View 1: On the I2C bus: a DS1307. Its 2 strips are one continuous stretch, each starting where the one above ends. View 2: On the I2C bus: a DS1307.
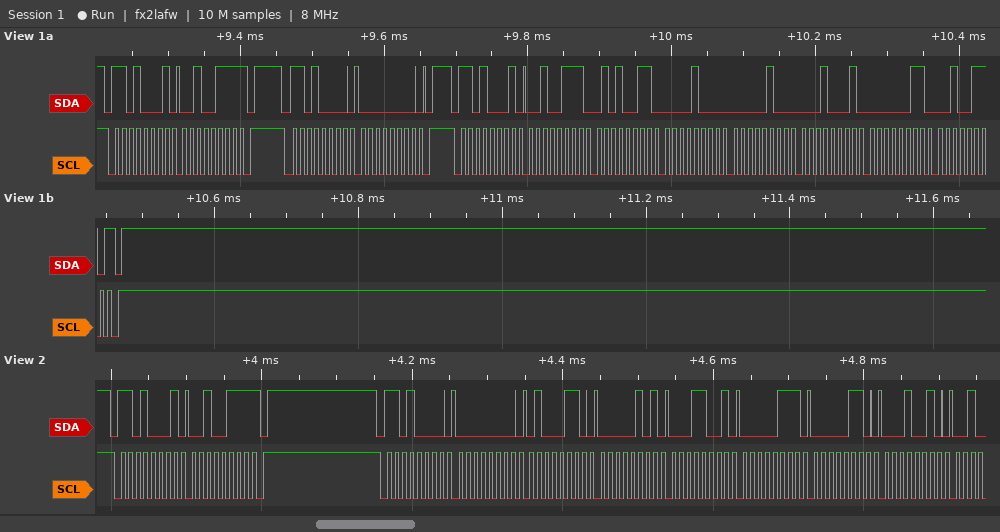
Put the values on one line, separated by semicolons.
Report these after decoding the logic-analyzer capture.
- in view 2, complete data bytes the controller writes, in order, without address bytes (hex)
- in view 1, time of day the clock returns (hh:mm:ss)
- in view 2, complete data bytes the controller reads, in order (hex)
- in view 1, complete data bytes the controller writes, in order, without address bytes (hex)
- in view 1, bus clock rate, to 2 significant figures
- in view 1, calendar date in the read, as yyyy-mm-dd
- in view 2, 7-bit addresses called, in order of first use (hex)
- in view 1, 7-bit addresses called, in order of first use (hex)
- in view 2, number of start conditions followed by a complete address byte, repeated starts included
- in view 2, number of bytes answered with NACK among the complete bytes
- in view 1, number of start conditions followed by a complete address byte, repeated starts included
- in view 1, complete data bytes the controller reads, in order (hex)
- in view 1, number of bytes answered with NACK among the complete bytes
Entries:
00 46 05 19 07 06 12; 08:53:27; 27; 00; 100 kHz; 2026-03-11; 0x68; 0x68; 2; 1; 3; 27 27 53 08 04 11 03 26; 2
